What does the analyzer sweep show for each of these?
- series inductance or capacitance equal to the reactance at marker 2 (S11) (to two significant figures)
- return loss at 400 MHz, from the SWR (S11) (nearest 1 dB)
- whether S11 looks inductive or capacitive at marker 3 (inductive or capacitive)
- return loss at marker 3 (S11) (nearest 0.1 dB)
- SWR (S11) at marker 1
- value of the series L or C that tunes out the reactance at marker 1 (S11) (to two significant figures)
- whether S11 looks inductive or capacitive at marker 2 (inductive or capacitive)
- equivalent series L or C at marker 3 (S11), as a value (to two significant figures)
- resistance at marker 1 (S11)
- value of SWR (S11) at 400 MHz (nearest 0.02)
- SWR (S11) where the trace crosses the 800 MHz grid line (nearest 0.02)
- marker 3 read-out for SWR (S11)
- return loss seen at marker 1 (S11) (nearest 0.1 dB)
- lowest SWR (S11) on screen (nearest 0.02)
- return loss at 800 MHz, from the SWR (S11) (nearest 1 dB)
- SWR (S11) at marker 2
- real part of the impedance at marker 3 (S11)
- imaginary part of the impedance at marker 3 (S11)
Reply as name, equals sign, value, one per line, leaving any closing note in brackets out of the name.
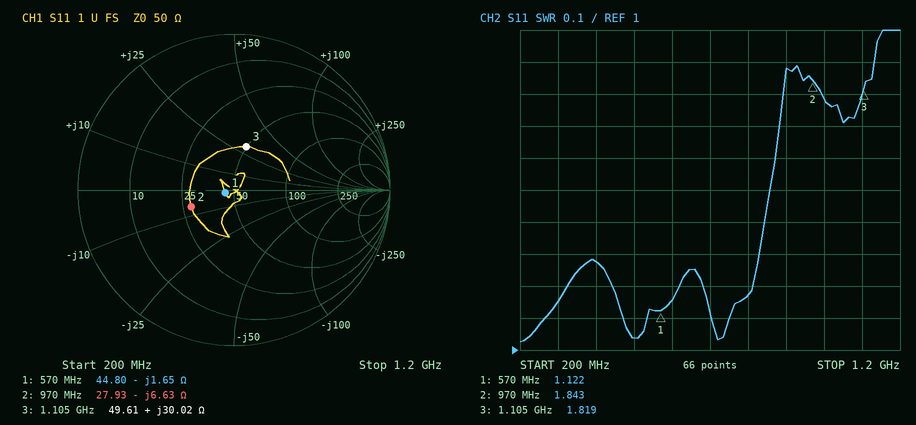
series inductance or capacitance equal to the reactance at marker 2 (S11) = 25 pF
return loss at 400 MHz, from the SWR (S11) = 18 dB
whether S11 looks inductive or capacitive at marker 3 = inductive
return loss at marker 3 (S11) = 10.8 dB
SWR (S11) at marker 1 = 1.122
value of the series L or C that tunes out the reactance at marker 1 (S11) = 460 pH
whether S11 looks inductive or capacitive at marker 2 = capacitive
equivalent series L or C at marker 3 (S11), as a value = 4.3 nH
resistance at marker 1 = 44.80 Ω
value of SWR (S11) at 400 MHz = 1.28
SWR (S11) where the trace crosses the 800 MHz grid line = 1.18
marker 3 read-out for SWR = 1.819
return loss seen at marker 1 (S11) = 24.8 dB
lowest SWR (S11) on screen = 1.02
return loss at 800 MHz, from the SWR (S11) = 22 dB
SWR (S11) at marker 2 = 1.843
real part of the impedance at marker 3 = 49.61 Ω
imaginary part of the impedance at marker 3 = +30.02 Ω
